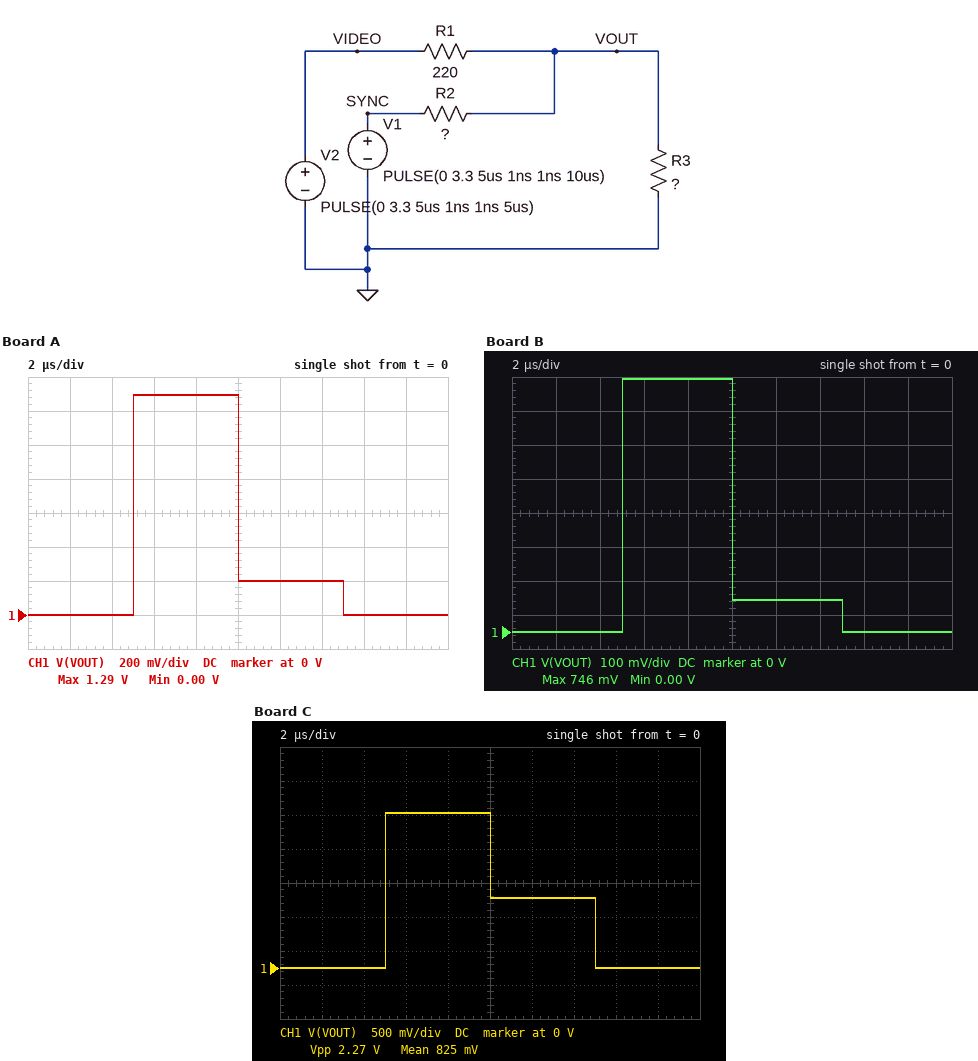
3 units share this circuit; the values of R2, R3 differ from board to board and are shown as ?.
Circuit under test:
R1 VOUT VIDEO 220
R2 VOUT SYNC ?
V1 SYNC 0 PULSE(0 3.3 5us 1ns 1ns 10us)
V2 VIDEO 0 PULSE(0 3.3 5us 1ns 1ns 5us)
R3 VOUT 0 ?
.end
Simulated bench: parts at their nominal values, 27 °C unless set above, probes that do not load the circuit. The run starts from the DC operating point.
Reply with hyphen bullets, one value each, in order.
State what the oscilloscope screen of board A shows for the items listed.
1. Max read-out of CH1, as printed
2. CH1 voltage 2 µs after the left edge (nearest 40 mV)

- 1.29 V
- 0 V
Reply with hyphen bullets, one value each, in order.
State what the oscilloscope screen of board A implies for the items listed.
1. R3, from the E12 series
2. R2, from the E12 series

- 120 Ω
- 1.2 kΩ
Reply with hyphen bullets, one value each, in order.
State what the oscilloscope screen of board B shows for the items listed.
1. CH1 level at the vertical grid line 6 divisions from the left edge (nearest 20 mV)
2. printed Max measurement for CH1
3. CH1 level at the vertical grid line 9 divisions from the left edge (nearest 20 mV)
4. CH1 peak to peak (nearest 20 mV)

- 100 mV
- 746 mV
- 0 V
- 740 mV
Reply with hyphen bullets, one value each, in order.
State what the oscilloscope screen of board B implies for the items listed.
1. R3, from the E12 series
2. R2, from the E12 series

- 56 Ω
- 1.5 kΩ
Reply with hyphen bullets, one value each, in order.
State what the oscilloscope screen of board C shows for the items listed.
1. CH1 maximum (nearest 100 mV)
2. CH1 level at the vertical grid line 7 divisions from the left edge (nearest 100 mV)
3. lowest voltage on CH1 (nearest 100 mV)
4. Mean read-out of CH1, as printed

- 2.3 V
- 1.0 V
- 0 V
- 825 mV
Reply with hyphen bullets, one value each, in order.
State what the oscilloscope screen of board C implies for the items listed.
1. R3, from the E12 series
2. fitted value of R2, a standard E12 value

- 270 Ω
- 270 Ω
